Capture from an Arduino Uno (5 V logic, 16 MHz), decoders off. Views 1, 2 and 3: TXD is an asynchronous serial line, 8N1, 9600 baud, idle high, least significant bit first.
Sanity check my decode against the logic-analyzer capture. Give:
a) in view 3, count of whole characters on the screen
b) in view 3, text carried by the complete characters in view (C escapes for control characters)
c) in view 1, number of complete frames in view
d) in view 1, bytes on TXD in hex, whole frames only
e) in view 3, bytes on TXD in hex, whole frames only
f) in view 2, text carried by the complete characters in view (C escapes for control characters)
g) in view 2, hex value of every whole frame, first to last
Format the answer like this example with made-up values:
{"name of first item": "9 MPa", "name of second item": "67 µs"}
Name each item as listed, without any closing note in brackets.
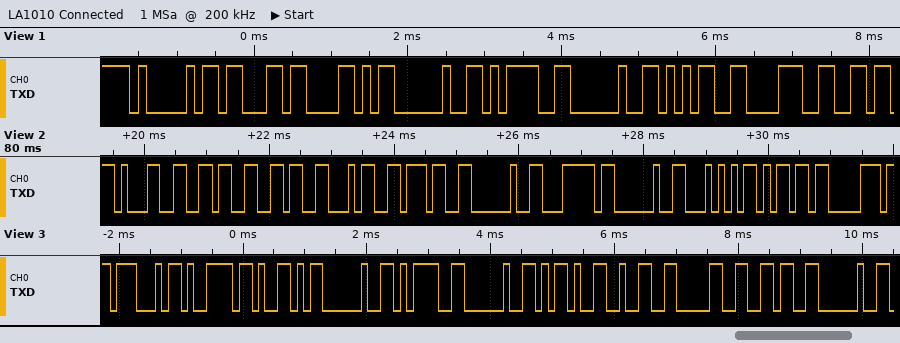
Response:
{"in view 3, count of whole characters on the screen": "11", "in view 3, text carried by the complete characters in view": "\"GyY = -206 \"", "in view 1, number of complete frames in view": "8", "in view 1, bytes on TXD in hex, whole frames only": "41 63 58 20 3D 20 35 38", "in view 3, bytes on TXD in hex, whole frames only": "47 79 59 20 3D 20 2D 32 30 36 20", "in view 2, text carried by the complete characters in view": "\"16647 | Tmp\"", "in view 2, hex value of every whole frame, first to last": "0x31 0x36 0x36 0x34 0x37 0x20 0x7C 0x20 0x54 0x6D 0x70"}
